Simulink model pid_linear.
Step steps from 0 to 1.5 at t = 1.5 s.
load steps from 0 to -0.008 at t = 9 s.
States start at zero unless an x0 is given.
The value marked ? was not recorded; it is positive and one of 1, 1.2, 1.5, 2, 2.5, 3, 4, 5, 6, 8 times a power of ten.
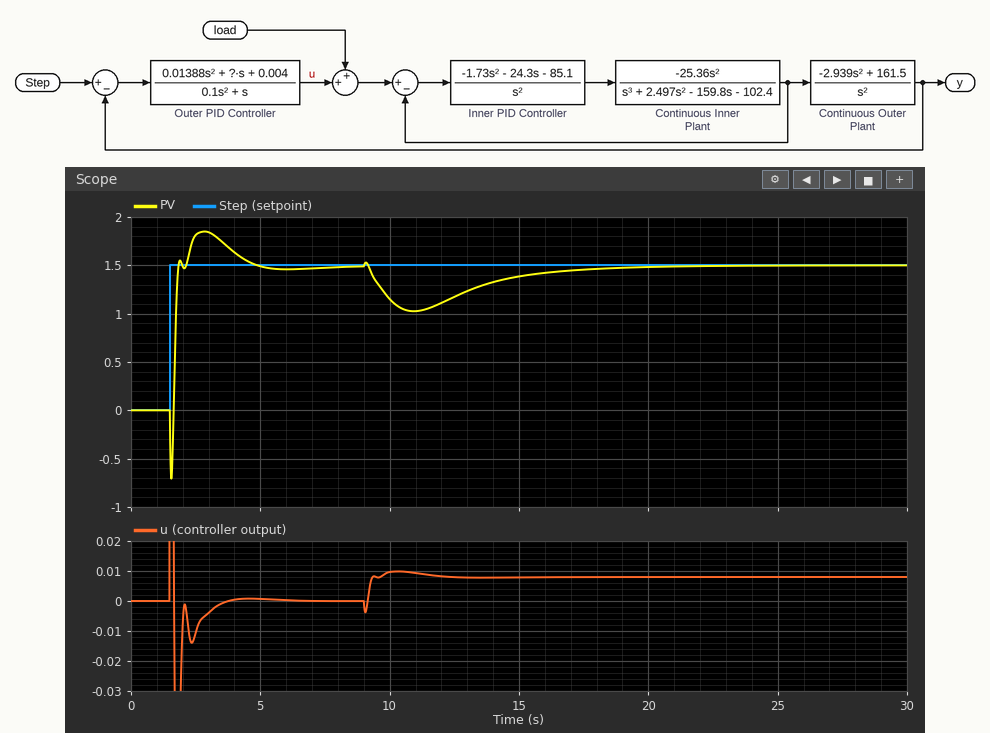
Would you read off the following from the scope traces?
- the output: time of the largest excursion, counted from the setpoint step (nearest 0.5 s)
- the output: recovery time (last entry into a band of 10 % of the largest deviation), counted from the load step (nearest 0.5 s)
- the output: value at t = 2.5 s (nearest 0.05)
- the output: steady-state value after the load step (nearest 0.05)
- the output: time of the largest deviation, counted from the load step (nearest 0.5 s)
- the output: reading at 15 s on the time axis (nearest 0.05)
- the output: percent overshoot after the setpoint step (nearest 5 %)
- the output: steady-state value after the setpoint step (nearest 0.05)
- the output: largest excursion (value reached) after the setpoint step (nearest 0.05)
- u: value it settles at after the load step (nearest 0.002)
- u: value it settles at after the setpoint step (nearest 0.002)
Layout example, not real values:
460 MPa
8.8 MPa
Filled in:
1.5 s
8.5 s
1.80
1.50
2.0 s
1.40
25 %
1.50
1.85
0.008
0.000
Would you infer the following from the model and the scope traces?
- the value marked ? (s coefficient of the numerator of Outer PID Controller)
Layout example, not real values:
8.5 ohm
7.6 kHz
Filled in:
0.015
